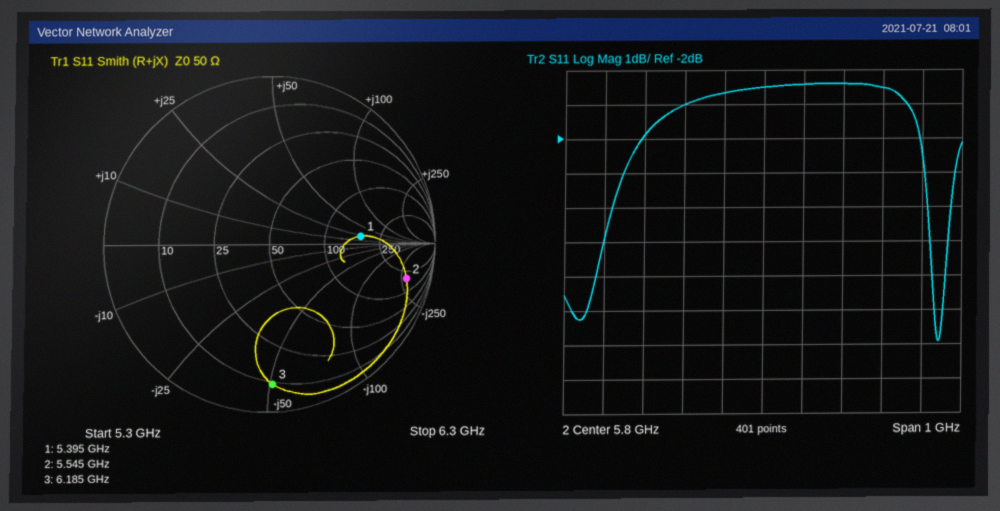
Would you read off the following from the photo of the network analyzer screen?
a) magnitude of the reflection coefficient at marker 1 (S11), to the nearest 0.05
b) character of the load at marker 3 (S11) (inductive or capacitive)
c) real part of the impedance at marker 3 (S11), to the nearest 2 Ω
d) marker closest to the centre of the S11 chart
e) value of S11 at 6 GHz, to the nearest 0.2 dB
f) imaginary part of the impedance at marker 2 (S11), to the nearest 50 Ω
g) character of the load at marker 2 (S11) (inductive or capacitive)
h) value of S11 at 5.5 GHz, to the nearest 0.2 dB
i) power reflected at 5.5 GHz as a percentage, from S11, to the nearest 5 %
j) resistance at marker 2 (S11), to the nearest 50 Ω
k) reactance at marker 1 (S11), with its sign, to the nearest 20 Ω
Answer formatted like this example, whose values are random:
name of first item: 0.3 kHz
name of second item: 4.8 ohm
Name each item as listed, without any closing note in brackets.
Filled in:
magnitude of the reflection coefficient at marker 1 (S11), to the nearest 0.05: 0.55
character of the load at marker 3 (S11): capacitive
real part of the impedance at marker 3 (S11), to the nearest 2 Ω: 10 Ω
marker closest to the centre of the S11 chart: marker 1
value of S11 at 6 GHz, to the nearest 0.2 dB: -0.4 dB
imaginary part of the impedance at marker 2 (S11), to the nearest 50 Ω: -300 Ω
character of the load at marker 2 (S11): capacitive
value of S11 at 5.5 GHz, to the nearest 0.2 dB: -1.8 dB
power reflected at 5.5 GHz as a percentage, from S11, to the nearest 5 %: 65 %
resistance at marker 2 (S11), to the nearest 50 Ω: 200 Ω
reactance at marker 1 (S11), with its sign, to the nearest 20 Ω: +20 Ω
